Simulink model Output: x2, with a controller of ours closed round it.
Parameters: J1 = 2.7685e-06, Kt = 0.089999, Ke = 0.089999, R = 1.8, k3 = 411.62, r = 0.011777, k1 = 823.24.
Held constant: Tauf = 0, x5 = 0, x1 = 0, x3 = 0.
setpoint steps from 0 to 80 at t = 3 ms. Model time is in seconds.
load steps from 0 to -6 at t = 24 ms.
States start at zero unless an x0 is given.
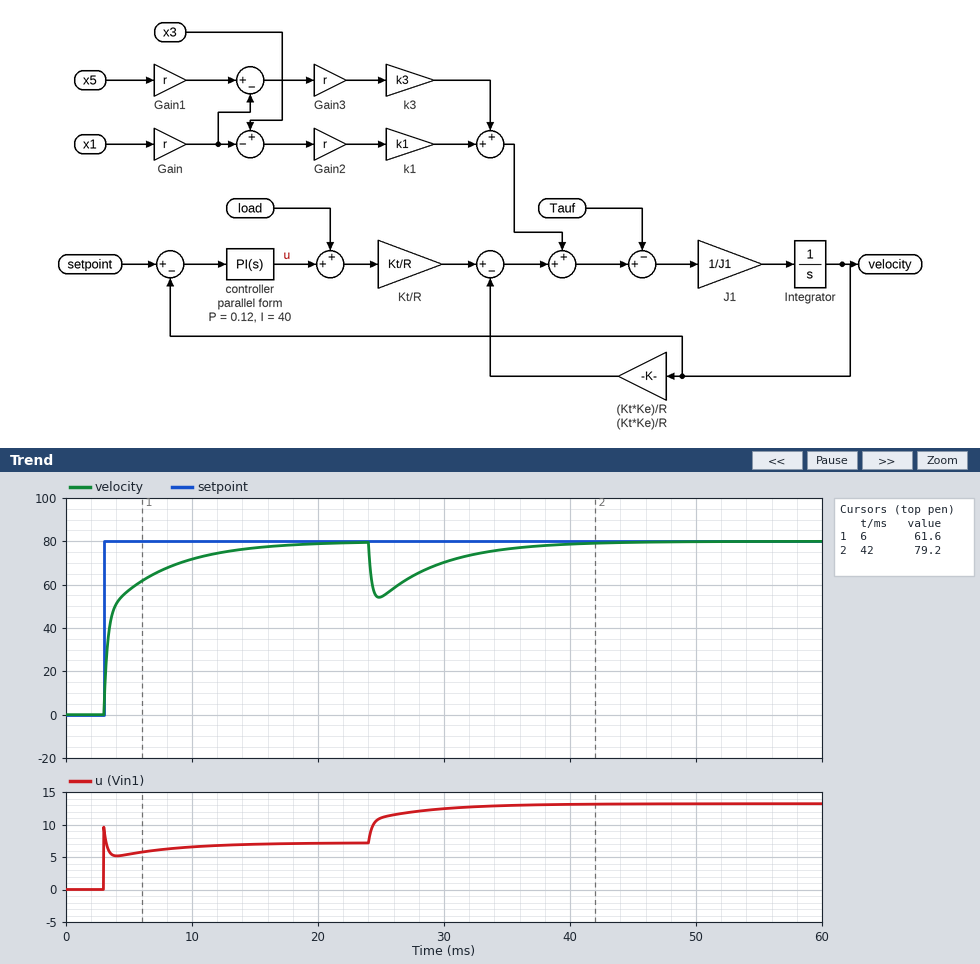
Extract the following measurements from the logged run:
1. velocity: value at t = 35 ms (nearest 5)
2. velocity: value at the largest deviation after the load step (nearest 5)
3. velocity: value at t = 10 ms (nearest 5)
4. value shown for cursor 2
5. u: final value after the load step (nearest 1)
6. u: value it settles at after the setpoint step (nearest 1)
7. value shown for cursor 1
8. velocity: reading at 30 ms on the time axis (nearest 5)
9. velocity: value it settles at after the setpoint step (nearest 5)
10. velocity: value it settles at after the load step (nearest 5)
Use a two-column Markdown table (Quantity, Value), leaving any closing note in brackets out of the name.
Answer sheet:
| Quantity | Value |
|---|---|
| velocity: value at t = 35 ms | 75 |
| velocity: value at the largest deviation after the load step | 55 |
| velocity: value at t = 10 ms | 70 |
| value shown for cursor 2 | 79.2 |
| u: final value after the load step | 13 |
| u: value it settles at after the setpoint step | 7 |
| value shown for cursor 1 | 61.6 |
| velocity: reading at 30 ms on the time axis | 70 |
| velocity: value it settles at after the setpoint step | 80 |
| velocity: value it settles at after the load step | 80 |
